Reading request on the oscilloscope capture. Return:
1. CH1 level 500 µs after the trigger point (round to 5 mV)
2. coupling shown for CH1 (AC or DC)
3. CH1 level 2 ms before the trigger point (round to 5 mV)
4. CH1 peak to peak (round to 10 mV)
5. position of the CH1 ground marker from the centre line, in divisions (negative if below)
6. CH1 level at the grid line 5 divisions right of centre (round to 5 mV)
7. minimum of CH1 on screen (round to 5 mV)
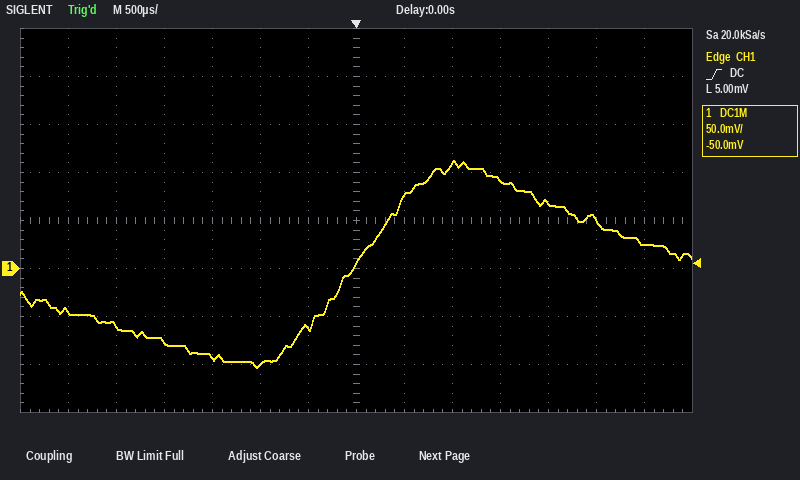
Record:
75 mV
DC
-75 mV
220 mV
-1.0 div
50 mV
-105 mV
